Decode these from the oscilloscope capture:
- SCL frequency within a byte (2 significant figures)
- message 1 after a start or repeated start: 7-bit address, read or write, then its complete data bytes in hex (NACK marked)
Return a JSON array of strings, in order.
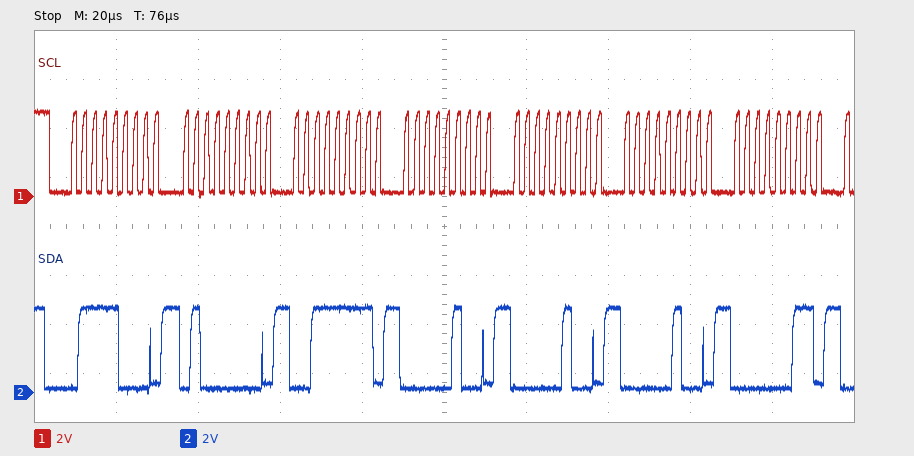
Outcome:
["400 kHz", "0x3C write: 40 3F 04 04 04 03"]
